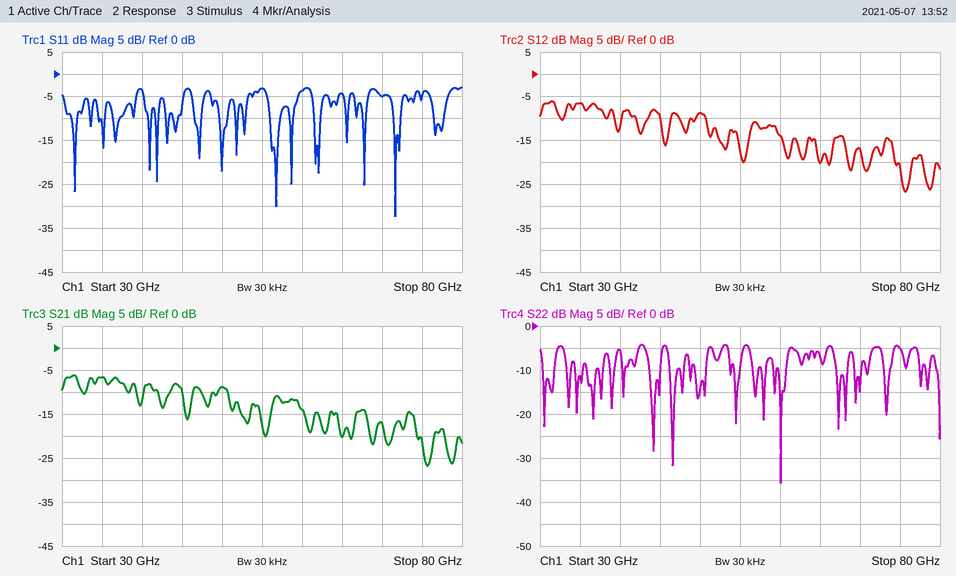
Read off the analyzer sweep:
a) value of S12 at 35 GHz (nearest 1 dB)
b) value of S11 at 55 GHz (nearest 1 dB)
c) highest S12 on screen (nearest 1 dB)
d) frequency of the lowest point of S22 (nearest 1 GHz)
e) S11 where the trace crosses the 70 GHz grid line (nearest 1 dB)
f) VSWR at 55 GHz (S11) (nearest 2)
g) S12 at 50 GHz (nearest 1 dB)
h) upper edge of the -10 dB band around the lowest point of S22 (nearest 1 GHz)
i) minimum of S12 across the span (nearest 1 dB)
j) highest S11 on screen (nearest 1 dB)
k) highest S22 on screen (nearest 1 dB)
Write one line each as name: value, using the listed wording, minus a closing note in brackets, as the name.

value of S12 at 35 GHz: -7 dB
value of S11 at 55 GHz: -3 dB
highest S12 on screen: -6 dB
frequency of the lowest point of S22: 60 GHz
S11 where the trace crosses the 70 GHz grid line: -5 dB
VSWR at 55 GHz (S11): 6
S12 at 50 GHz: -9 dB
upper edge of the -10 dB band around the lowest point of S22: 61 GHz
minimum of S12 across the span: -27 dB
highest S11 on screen: -3 dB
highest S22 on screen: -4 dB
